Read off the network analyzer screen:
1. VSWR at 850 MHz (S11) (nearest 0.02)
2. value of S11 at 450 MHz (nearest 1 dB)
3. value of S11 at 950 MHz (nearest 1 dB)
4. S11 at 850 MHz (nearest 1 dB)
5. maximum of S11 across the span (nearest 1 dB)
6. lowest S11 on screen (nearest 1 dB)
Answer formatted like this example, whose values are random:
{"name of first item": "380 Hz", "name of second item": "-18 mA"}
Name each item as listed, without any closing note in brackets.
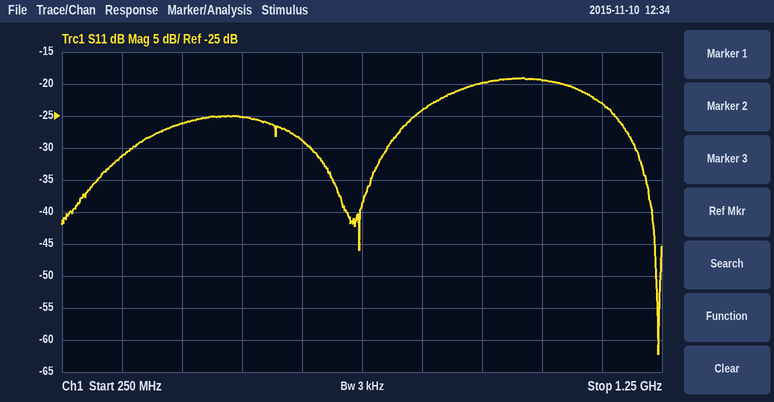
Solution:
{"VSWR at 850 MHz (S11)": "1.14", "value of S11 at 450 MHz": "-26 dB", "value of S11 at 950 MHz": "-20 dB", "S11 at 850 MHz": "-24 dB", "maximum of S11 across the span": "-19 dB", "lowest S11 on screen": "-62 dB"}
